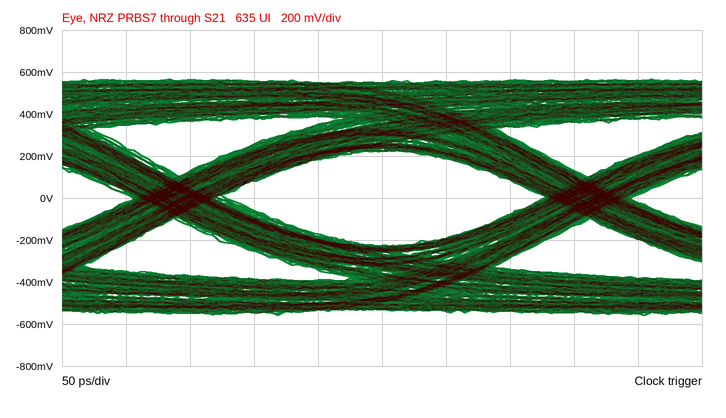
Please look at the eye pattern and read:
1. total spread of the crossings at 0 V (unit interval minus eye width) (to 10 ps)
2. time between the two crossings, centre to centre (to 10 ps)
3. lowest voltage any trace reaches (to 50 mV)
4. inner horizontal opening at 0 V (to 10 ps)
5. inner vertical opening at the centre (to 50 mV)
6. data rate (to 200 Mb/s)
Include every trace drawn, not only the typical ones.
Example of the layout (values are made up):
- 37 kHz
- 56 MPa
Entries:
- 70 ps
- 320 ps
- -550 mV
- 250 ps
- 450 mV
- 3.2 Gb/s
